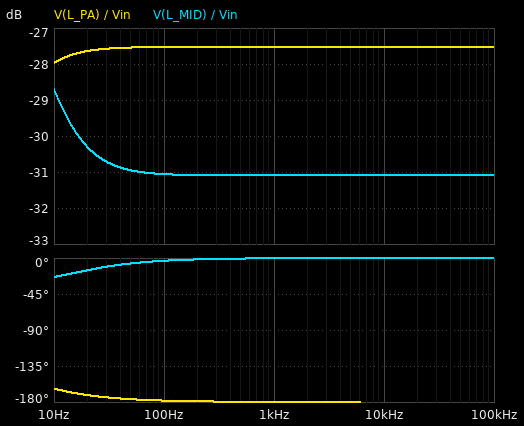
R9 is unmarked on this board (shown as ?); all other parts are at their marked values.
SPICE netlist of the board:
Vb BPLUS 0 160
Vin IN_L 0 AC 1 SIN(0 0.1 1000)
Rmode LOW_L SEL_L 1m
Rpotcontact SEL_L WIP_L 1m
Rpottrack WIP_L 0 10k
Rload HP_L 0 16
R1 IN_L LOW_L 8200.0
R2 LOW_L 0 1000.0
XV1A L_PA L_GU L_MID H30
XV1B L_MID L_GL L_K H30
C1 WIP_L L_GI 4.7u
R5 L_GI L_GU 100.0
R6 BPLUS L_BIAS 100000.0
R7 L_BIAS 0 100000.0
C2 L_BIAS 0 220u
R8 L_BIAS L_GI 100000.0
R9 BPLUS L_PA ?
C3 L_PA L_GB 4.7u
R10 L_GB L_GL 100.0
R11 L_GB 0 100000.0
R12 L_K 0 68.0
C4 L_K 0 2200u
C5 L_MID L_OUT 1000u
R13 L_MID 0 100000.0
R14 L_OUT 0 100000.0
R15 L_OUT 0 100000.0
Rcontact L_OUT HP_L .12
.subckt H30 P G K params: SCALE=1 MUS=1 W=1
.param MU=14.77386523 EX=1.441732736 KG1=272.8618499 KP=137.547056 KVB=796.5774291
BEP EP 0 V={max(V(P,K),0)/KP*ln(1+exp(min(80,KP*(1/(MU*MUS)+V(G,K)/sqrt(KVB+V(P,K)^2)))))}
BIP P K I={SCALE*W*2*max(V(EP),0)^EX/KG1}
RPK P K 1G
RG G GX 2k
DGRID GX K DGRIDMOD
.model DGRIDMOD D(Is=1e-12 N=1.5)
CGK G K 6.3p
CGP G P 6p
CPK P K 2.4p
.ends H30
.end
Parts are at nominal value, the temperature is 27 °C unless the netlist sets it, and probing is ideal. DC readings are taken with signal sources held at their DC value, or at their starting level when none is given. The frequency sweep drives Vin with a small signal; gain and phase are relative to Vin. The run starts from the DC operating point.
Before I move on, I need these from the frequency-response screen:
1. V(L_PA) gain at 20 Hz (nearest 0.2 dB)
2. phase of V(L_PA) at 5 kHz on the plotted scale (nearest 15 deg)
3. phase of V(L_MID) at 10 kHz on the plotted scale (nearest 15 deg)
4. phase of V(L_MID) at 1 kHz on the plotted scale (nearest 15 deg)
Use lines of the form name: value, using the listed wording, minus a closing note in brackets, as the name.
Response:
V(L_PA) gain at 20 Hz: -27.6 dB
phase of V(L_PA) at 5 kHz on the plotted scale: -180 deg
phase of V(L_MID) at 10 kHz on the plotted scale: 0 deg
phase of V(L_MID) at 1 kHz on the plotted scale: 0 deg
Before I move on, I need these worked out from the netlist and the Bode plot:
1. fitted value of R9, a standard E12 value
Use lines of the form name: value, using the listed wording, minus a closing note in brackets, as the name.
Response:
fitted value of R9, a standard E12 value: 39 Ω
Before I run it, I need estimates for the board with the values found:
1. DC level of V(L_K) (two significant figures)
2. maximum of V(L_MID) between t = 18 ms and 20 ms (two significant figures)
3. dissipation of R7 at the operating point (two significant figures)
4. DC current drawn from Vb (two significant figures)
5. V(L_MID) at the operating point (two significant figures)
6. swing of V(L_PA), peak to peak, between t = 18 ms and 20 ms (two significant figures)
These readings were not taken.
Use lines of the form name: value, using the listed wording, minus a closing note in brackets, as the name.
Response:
DC level of V(L_K): 2.5 V
maximum of V(L_MID) between t = 18 ms and 20 ms: 82 V
dissipation of R7 at the operating point: 64 mW
DC current drawn from Vb: 38 mA
V(L_MID) at the operating point: 82 V
swing of V(L_PA), peak to peak, between t = 18 ms and 20 ms: 8.4 mV
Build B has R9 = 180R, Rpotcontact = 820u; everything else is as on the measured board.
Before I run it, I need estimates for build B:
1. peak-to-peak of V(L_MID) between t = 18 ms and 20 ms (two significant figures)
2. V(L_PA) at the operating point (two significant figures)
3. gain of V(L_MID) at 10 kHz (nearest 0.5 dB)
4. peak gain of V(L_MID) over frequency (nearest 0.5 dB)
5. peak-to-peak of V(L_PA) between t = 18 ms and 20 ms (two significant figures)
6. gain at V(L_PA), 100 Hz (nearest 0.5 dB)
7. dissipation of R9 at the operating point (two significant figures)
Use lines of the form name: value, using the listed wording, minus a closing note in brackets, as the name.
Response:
peak-to-peak of V(L_MID) between t = 18 ms and 20 ms: 8.7 mV
V(L_PA) at the operating point: 150 V
gain of V(L_MID) at 10 kHz: -27.0 dB
peak gain of V(L_MID) over frequency: -22.0 dB
peak-to-peak of V(L_PA) between t = 18 ms and 20 ms: 25 mV
gain at V(L_PA), 100 Hz: -18.0 dB
dissipation of R9 at the operating point: 250 mW
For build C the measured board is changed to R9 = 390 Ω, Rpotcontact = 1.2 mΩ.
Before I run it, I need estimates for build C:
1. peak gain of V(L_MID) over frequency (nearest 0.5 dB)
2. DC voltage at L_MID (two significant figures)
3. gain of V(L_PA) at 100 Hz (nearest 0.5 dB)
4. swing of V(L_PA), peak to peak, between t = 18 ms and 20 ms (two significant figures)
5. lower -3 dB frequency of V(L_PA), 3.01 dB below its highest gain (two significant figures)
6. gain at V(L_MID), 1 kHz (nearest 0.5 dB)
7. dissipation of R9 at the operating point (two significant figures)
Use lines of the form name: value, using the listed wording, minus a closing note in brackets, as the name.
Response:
peak gain of V(L_MID) over frequency: -22.0 dB
DC voltage at L_MID: 81 V
gain of V(L_PA) at 100 Hz: -15.0 dB
swing of V(L_PA), peak to peak, between t = 18 ms and 20 ms: 36 mV
lower -3 dB frequency of V(L_PA), 3.01 dB below its highest gain: 5.7 Hz
gain at V(L_MID), 1 kHz: -25.5 dB
dissipation of R9 at the operating point: 530 mW
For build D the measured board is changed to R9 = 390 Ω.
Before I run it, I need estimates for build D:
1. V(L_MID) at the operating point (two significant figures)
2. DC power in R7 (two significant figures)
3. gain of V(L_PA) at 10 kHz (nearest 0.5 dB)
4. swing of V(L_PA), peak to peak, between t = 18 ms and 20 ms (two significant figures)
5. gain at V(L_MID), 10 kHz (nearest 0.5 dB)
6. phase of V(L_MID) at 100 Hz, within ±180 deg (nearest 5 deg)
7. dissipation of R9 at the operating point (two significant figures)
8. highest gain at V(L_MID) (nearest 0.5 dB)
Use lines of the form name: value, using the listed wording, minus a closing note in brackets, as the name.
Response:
V(L_MID) at the operating point: 81 V
DC power in R7: 64 mW
gain of V(L_PA) at 10 kHz: -15.0 dB
swing of V(L_PA), peak to peak, between t = 18 ms and 20 ms: 36 mV
gain at V(L_MID), 10 kHz: -25.5 dB
phase of V(L_MID) at 100 Hz, within ±180 deg: 0 deg
dissipation of R9 at the operating point: 530 mW
highest gain at V(L_MID): -22.0 dB
